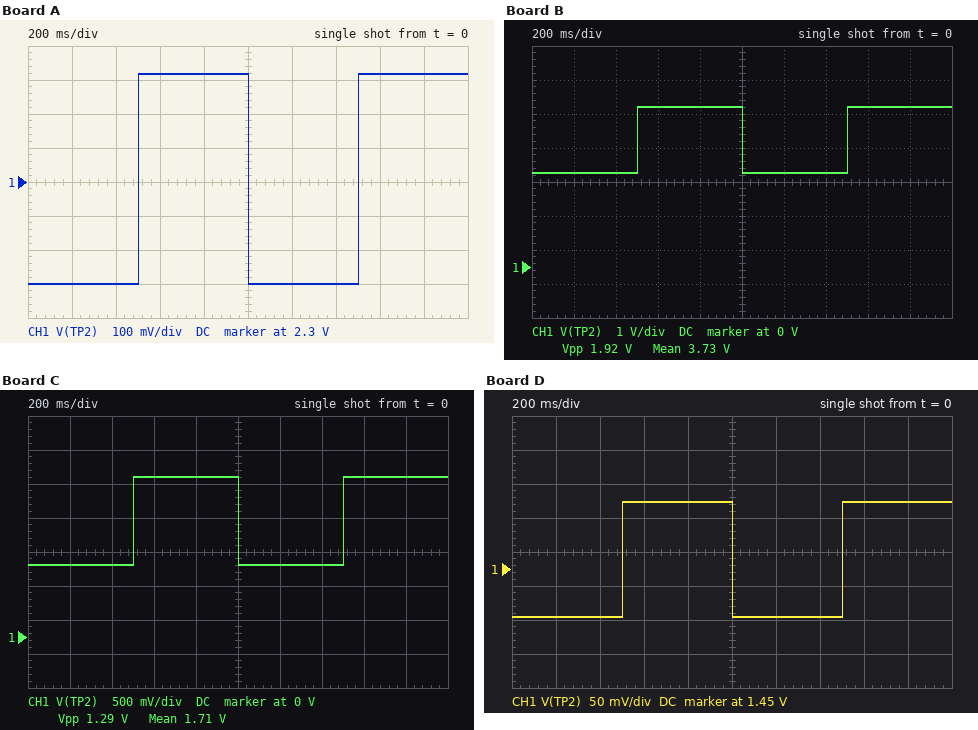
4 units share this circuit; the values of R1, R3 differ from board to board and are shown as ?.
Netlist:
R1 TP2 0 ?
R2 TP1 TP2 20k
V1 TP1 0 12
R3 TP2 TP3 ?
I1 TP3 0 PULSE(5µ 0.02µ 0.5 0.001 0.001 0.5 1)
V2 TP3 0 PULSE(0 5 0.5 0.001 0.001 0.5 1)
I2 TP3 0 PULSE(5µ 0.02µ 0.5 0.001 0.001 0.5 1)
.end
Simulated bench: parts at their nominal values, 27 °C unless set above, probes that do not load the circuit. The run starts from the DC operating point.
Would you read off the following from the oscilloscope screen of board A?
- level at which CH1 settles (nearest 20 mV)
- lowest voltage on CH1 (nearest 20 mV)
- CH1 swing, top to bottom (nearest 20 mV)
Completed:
2.62 V
2.00 V
620 mV
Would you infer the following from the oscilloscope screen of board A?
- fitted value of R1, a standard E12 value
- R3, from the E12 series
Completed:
4.7 kΩ
27 kΩ
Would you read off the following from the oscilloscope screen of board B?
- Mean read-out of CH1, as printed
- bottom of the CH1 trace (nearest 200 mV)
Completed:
3.73 V
2.8 V
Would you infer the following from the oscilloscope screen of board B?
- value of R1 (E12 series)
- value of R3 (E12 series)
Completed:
12 kΩ
12 kΩ
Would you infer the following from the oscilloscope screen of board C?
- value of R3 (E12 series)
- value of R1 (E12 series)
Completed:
6.8 kΩ
2.7 kΩ
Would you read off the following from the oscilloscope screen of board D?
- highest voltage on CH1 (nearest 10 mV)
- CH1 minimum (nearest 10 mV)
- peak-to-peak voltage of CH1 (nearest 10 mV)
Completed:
1.55 V
1.38 V
170 mV
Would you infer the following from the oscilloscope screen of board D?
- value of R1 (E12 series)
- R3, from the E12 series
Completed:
2.7 kΩ
68 kΩ
